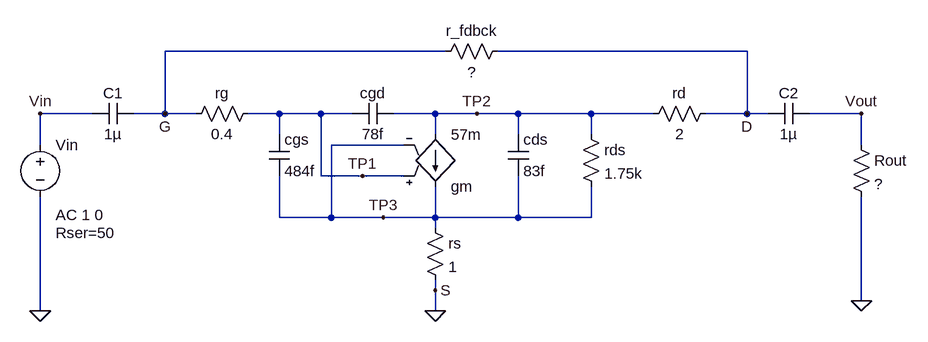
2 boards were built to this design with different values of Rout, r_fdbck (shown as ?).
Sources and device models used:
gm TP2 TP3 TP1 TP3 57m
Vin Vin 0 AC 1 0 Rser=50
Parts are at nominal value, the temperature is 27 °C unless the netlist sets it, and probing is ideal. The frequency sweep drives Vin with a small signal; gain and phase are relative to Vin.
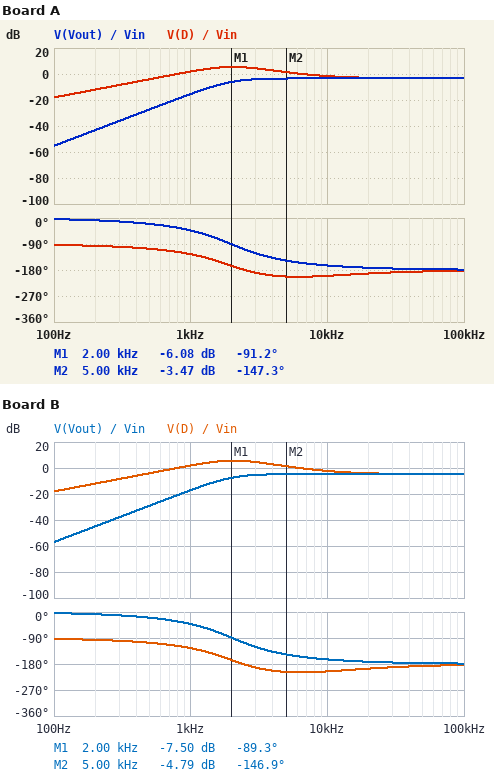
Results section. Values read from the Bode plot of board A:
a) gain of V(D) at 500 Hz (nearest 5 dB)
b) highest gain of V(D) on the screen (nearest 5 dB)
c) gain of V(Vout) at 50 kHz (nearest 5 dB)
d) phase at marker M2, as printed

-5 dB
5 dB
-5 dB
-147.3 deg
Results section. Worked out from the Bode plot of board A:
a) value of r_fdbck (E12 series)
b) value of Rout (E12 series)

220 Ω
22 Ω
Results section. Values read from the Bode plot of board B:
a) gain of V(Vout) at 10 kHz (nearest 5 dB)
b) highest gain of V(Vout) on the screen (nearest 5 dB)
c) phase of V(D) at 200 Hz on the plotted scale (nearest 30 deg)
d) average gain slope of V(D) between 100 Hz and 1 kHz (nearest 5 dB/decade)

-5 dB
-5 dB
-90 deg
20 dB/decade
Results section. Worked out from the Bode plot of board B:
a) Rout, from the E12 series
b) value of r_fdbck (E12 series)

18 Ω
220 Ω
